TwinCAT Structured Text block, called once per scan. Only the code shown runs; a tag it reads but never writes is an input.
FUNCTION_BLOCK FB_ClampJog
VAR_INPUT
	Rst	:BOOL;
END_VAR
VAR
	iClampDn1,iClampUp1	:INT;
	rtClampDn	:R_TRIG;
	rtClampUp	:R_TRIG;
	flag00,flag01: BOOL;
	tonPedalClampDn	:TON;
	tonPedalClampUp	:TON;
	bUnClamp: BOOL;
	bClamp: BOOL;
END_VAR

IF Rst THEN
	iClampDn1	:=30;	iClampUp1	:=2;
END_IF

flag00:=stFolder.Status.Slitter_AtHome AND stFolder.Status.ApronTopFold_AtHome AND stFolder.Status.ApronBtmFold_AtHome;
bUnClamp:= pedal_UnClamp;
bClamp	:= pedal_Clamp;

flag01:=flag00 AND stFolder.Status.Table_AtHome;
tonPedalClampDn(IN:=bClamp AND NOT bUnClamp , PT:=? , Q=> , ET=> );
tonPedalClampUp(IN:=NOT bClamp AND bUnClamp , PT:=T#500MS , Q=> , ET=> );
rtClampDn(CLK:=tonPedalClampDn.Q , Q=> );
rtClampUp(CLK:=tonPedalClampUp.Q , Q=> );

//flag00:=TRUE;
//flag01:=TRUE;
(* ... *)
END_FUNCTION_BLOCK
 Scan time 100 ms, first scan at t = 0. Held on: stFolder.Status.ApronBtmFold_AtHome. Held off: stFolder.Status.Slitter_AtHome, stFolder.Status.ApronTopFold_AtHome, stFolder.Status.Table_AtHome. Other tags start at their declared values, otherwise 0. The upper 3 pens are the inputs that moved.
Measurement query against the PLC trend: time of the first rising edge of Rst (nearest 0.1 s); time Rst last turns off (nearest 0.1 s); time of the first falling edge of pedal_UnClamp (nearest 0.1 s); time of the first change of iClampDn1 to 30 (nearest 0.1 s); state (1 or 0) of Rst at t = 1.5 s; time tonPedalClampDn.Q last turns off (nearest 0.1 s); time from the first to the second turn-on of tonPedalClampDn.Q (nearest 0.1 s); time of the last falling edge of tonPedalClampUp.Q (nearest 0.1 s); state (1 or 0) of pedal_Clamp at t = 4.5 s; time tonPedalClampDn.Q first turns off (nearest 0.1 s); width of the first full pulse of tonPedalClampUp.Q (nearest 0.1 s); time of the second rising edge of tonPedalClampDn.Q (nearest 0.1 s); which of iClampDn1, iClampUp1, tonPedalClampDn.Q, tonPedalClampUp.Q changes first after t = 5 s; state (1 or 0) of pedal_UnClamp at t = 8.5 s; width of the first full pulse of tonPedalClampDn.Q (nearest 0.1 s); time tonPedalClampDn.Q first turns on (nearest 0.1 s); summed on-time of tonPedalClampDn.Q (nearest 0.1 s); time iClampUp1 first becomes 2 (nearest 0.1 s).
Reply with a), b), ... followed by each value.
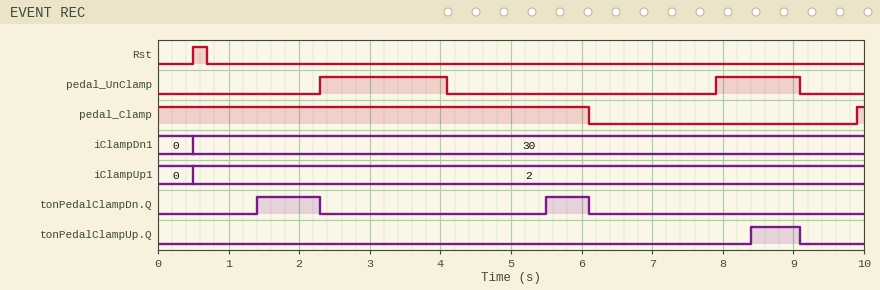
a) 0.5 s
b) 0.7 s
c) 4.1 s
d) 0.5 s
e) 0
f) 6.1 s
g) 4.1 s
h) 9.1 s
i) 1
j) 2.3 s
k) 0.7 s
l) 5.5 s
m) tonPedalClampDn.Q
n) 1
o) 0.9 s
p) 1.4 s
q) 1.5 s
r) 0.5 s
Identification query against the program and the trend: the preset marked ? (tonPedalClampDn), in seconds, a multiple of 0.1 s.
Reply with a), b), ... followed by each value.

a) 1.4 s
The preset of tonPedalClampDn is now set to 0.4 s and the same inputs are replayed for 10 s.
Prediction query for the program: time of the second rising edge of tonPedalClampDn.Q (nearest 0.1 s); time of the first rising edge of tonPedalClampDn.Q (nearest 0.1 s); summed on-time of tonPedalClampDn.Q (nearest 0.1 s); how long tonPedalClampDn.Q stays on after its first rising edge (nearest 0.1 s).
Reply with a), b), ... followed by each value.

a) 4.5 s
b) 0.4 s
c) 3.5 s
d) 1.9 s
